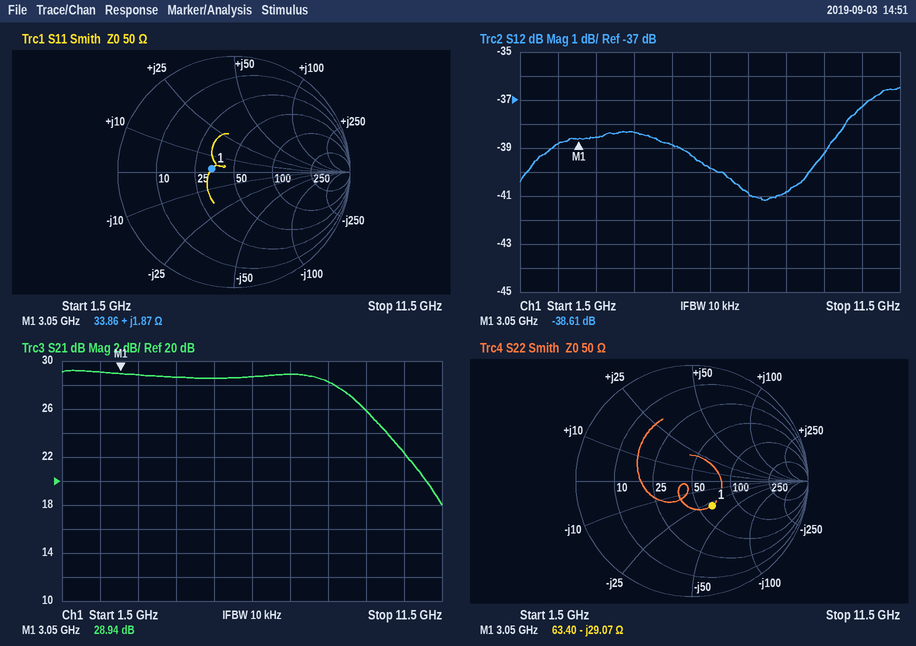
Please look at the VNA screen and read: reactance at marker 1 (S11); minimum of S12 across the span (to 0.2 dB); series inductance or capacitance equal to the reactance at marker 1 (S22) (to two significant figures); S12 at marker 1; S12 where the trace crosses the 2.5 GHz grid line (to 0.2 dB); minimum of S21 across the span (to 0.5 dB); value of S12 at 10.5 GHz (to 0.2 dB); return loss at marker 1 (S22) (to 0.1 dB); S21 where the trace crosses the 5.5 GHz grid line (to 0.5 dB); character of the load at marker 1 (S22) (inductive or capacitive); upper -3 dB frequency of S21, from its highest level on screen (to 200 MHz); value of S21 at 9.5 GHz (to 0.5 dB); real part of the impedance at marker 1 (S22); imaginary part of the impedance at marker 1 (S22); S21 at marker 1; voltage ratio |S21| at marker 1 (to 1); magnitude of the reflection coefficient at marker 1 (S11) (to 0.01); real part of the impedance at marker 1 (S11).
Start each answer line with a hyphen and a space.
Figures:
- +1.87 Ω
- -41.2 dB
- 1.8 pF
- -38.61 dB
- -38.8 dB
- 18.0 dB
- -37.2 dB
- 11.3 dB
- 28.5 dB
- capacitive
- 9.4 GHz
- 26.0 dB
- 63.40 Ω
- -29.07 Ω
- 28.94 dB
- 28
- 0.19
- 33.86 Ω
